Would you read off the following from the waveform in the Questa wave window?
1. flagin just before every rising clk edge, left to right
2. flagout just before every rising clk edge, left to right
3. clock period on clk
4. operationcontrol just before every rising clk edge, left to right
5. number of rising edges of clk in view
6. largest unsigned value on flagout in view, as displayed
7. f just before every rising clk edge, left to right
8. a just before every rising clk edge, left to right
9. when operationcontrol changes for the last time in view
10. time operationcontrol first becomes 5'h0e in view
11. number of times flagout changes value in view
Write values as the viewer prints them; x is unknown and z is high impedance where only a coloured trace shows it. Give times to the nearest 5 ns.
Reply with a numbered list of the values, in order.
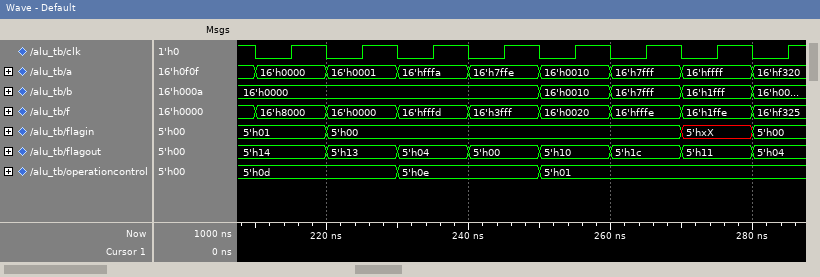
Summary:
1. 5'h01, 5'h00, 5'h00, 5'h00, 5'h00, 5'h00, 5'hxX, 5'h00
2. 5'h14, 5'h13, 5'h04, 5'h00, 5'h10, 5'h1c, 5'h11, 5'h04
3. 10 ns
4. 5'h0d, 5'h0d, 5'h0e, 5'h0e, 5'h01, 5'h01, 5'h01, 5'h01
5. 8
6. 5'h1c
7. 16'h8000, 16'h0000, 16'hfffd, 16'h3fff, 16'h0020, 16'hfffe, 16'h1ffe, 16'hf325
8. 16'h0000, 16'h0001, 16'hfffa, 16'h7ffe, 16'h0010, 16'h7fff, 16'hffff, 16'hf320
9. 250 ns
10. 230 ns
11. 7
